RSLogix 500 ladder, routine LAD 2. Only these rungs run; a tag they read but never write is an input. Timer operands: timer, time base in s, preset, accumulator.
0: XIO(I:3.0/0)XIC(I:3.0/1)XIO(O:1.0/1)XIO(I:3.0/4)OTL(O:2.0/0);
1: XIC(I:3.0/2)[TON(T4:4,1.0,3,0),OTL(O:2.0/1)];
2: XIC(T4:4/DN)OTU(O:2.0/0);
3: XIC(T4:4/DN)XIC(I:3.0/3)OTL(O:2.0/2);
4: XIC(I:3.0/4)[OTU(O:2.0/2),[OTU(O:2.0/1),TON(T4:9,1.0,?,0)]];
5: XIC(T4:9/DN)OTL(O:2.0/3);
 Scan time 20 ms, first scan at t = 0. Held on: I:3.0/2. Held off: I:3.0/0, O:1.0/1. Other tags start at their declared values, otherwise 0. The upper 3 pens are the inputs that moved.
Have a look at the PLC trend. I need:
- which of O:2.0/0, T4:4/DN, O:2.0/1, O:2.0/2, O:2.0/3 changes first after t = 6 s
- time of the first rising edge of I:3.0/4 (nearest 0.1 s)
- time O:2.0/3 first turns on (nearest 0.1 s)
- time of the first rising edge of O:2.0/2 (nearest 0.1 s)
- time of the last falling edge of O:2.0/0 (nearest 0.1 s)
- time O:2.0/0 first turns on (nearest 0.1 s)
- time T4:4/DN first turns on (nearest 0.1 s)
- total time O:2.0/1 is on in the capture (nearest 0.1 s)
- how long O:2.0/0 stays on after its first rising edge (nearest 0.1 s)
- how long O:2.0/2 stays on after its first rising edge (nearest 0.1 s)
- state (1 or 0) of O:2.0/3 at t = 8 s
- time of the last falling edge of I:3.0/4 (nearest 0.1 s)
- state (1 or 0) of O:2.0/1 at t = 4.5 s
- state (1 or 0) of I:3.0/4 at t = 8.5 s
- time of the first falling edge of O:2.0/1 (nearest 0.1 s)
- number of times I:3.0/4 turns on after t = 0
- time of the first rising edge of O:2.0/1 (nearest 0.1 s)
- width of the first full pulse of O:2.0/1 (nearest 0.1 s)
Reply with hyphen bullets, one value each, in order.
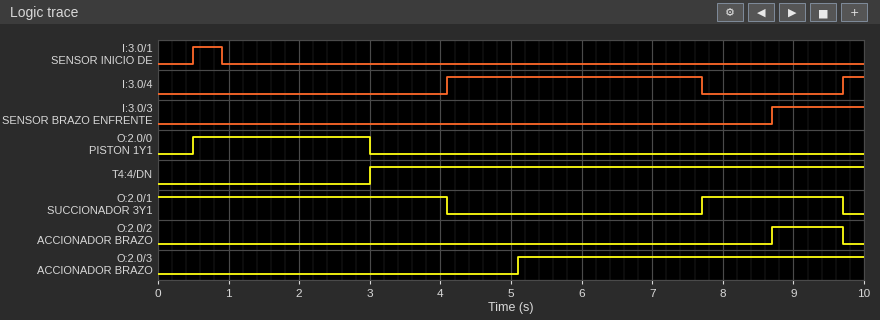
- O:2.0/1
- 4.1 s
- 5.1 s
- 8.7 s
- 3.0 s
- 0.5 s
- 3.0 s
- 6.1 s
- 2.5 s
- 1.0 s
- 1
- 7.7 s
- 0
- 0
- 4.1 s
- 2
- 7.7 s
- 2.0 s
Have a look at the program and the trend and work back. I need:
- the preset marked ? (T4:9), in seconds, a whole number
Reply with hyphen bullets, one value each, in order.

- 1 s
